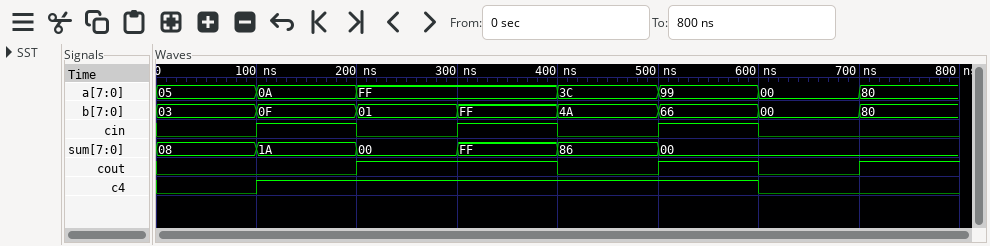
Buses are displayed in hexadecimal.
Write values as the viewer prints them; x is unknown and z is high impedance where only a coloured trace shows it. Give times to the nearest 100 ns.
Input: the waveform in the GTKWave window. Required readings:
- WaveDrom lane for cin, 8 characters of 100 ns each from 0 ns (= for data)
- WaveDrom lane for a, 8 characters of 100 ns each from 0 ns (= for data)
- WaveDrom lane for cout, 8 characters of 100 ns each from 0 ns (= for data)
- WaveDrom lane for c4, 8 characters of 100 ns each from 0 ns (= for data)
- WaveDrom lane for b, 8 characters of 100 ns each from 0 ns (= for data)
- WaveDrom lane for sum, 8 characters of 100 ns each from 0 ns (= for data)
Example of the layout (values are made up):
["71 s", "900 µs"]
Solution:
["{name: 'cin', wave: '0101010.'}", "{name: 'a', wave: '===.====', data: '05 0A FF 3C 99 00 80'}", "{name: 'cout', wave: '0.1.0101'}", "{name: 'c4', wave: '01....0.'}", "{name: 'b', wave: '========', data: '03 0F 01 FF 4A 66 00 80'}", "{name: 'sum', wave: '======..', data: '08 1A 00 FF 86 00'}"]
